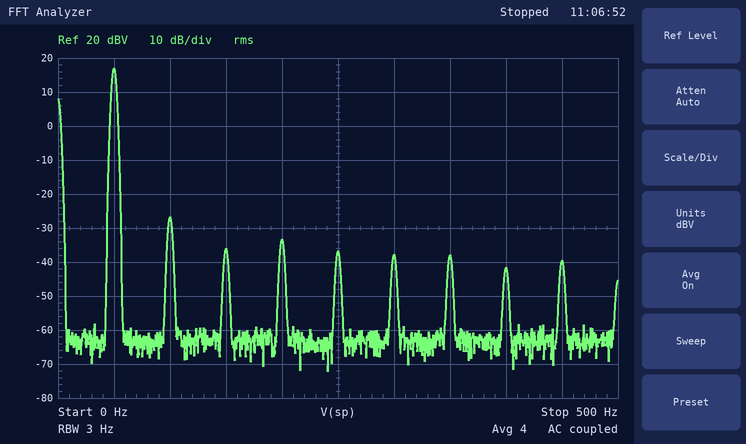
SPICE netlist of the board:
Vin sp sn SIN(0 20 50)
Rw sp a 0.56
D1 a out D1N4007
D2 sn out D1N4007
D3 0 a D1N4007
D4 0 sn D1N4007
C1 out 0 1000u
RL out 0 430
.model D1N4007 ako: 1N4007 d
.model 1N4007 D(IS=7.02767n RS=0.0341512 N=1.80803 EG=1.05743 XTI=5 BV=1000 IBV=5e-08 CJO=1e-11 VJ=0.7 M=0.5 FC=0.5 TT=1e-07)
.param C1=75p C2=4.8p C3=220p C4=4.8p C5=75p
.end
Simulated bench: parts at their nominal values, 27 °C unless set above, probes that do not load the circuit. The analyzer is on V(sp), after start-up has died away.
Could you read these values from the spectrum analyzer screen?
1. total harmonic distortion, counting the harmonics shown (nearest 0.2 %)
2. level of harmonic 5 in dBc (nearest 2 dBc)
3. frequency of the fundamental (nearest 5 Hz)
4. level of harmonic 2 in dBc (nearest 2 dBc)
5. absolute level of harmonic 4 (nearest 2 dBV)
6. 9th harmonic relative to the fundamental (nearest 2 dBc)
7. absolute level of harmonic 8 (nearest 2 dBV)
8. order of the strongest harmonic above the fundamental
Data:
0.8 %
-54 dBc
50 Hz
-44 dBc
-34 dBV
-56 dBc
-42 dBV
2
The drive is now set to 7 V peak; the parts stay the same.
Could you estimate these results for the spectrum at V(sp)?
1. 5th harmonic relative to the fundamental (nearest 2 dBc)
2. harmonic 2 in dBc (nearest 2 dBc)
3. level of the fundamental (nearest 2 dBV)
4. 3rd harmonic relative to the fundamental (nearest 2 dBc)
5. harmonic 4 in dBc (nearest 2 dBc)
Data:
-56 dBc
-46 dBc
8 dBV
-54 dBc
-52 dBc
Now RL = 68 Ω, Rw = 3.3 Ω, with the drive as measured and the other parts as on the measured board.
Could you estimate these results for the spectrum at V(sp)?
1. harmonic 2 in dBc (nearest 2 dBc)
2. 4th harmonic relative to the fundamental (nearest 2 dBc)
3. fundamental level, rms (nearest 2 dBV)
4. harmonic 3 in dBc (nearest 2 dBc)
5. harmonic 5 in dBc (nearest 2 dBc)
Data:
-30 dBc
-40 dBc
18 dBV
-26 dBc
-32 dBc
